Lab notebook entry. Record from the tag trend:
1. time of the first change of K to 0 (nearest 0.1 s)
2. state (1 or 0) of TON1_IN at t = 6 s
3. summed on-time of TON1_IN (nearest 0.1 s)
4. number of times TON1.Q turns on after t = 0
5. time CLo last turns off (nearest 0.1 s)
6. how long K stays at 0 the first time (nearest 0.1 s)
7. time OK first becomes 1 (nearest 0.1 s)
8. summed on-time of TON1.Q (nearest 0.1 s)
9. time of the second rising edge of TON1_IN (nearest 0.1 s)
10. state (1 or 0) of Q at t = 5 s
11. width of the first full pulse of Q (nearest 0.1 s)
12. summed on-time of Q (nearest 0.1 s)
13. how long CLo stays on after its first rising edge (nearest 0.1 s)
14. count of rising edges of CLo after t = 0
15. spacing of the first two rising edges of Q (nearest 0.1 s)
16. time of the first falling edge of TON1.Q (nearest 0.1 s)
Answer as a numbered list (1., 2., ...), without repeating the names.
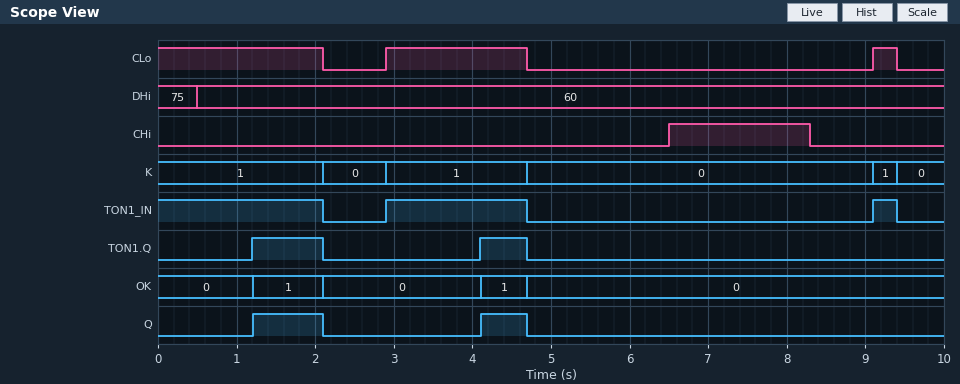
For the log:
1. 2.1 s
2. 0
3. 4.2 s
4. 2
5. 9.4 s
6. 0.8 s
7. 1.2 s
8. 1.5 s
9. 9.1 s
10. 0
11. 0.9 s
12. 1.5 s
13. 1.8 s
14. 2
15. 2.9 s
16. 2.1 s
